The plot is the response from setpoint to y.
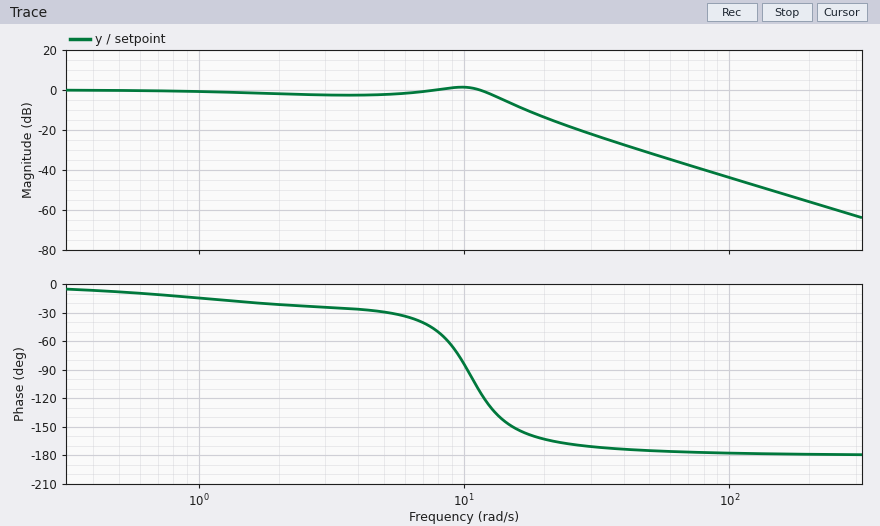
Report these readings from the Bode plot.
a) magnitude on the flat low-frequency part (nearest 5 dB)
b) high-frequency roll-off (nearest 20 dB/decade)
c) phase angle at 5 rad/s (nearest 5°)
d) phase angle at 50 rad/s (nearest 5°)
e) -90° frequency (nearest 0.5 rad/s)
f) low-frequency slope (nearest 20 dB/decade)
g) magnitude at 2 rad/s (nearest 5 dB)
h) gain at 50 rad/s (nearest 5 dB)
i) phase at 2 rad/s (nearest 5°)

0 dB
-40 dB/decade
-30°
-175°
10.5 rad/s
0 dB/decade
0 dB
-30 dB
-20°
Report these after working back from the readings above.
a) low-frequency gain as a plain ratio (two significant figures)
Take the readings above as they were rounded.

1.0
